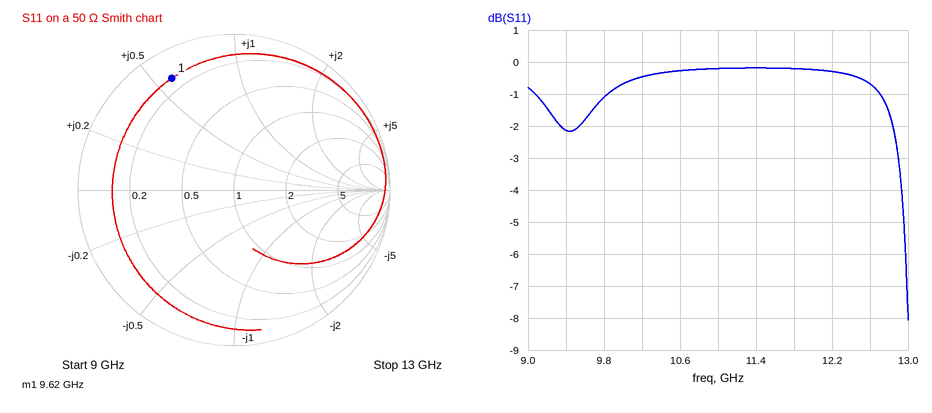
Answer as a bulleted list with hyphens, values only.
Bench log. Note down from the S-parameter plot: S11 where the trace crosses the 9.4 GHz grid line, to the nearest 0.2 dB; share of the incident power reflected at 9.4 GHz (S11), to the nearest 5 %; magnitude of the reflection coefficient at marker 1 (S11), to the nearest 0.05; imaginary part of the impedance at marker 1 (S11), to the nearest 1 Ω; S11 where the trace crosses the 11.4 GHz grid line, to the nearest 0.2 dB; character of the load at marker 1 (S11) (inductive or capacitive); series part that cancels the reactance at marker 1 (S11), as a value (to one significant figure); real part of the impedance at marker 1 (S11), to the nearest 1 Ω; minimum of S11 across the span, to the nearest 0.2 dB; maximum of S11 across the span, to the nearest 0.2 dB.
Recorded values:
- -2.2 dB
- 60 %
- 0.80
- +29 Ω
- -0.2 dB
- inductive
- 600 fF
- 7 Ω
- -8.0 dB
- -0.2 dB
